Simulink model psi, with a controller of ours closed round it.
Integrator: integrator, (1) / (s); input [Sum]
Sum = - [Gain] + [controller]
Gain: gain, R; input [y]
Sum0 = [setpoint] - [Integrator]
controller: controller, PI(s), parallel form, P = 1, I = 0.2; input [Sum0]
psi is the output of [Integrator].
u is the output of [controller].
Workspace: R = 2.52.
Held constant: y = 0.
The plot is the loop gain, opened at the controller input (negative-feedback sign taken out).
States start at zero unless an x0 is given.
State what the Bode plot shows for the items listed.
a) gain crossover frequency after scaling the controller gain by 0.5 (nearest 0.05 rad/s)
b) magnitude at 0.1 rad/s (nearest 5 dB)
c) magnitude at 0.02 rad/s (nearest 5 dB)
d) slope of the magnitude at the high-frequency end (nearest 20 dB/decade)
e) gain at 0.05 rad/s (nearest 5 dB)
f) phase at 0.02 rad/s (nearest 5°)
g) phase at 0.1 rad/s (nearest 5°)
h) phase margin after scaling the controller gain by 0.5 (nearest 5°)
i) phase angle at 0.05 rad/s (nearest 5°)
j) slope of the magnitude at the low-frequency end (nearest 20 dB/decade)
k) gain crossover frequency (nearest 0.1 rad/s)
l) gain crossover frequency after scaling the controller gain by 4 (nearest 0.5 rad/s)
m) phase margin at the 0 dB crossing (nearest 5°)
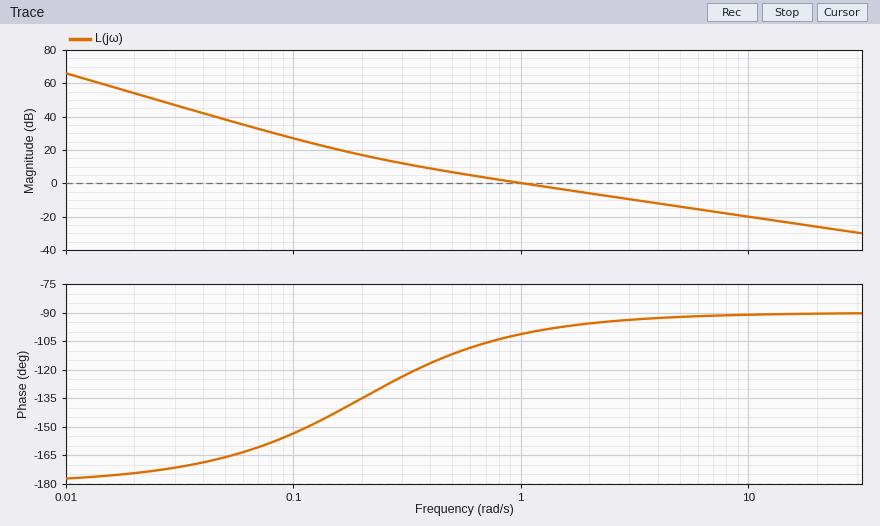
0.55 rad/s
25 dB
55 dB
-20 dB/decade
40 dB
-175°
-155°
70°
-165°
-40 dB/decade
1.0 rad/s
4.0 rad/s
80°
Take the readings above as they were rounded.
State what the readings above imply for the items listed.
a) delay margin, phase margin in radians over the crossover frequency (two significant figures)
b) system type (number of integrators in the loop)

1.4 s
2
